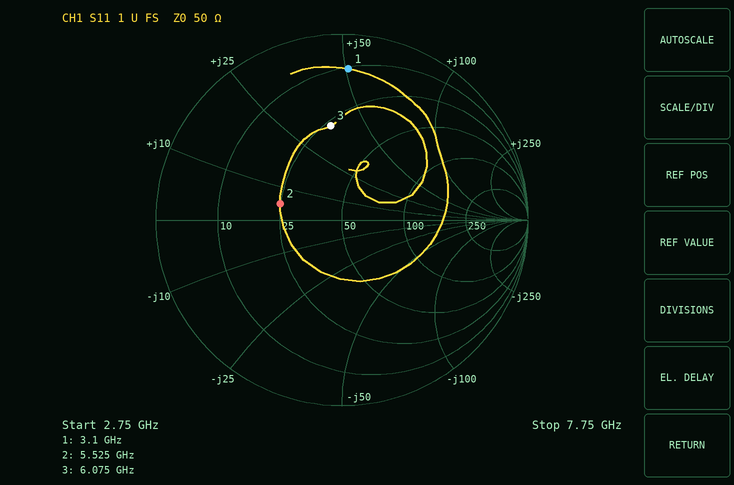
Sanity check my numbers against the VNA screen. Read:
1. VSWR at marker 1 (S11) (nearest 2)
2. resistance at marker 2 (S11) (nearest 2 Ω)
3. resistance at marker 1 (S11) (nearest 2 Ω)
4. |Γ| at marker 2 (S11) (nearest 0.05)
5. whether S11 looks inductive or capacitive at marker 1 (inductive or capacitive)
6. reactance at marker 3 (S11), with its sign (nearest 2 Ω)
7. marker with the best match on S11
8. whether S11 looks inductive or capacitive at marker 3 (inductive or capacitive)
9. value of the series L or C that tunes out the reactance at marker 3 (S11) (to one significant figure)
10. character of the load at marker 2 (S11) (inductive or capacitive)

10
24 Ω
10 Ω
0.35
inductive
+36 Ω
marker 2
inductive
700 fF
inductive
